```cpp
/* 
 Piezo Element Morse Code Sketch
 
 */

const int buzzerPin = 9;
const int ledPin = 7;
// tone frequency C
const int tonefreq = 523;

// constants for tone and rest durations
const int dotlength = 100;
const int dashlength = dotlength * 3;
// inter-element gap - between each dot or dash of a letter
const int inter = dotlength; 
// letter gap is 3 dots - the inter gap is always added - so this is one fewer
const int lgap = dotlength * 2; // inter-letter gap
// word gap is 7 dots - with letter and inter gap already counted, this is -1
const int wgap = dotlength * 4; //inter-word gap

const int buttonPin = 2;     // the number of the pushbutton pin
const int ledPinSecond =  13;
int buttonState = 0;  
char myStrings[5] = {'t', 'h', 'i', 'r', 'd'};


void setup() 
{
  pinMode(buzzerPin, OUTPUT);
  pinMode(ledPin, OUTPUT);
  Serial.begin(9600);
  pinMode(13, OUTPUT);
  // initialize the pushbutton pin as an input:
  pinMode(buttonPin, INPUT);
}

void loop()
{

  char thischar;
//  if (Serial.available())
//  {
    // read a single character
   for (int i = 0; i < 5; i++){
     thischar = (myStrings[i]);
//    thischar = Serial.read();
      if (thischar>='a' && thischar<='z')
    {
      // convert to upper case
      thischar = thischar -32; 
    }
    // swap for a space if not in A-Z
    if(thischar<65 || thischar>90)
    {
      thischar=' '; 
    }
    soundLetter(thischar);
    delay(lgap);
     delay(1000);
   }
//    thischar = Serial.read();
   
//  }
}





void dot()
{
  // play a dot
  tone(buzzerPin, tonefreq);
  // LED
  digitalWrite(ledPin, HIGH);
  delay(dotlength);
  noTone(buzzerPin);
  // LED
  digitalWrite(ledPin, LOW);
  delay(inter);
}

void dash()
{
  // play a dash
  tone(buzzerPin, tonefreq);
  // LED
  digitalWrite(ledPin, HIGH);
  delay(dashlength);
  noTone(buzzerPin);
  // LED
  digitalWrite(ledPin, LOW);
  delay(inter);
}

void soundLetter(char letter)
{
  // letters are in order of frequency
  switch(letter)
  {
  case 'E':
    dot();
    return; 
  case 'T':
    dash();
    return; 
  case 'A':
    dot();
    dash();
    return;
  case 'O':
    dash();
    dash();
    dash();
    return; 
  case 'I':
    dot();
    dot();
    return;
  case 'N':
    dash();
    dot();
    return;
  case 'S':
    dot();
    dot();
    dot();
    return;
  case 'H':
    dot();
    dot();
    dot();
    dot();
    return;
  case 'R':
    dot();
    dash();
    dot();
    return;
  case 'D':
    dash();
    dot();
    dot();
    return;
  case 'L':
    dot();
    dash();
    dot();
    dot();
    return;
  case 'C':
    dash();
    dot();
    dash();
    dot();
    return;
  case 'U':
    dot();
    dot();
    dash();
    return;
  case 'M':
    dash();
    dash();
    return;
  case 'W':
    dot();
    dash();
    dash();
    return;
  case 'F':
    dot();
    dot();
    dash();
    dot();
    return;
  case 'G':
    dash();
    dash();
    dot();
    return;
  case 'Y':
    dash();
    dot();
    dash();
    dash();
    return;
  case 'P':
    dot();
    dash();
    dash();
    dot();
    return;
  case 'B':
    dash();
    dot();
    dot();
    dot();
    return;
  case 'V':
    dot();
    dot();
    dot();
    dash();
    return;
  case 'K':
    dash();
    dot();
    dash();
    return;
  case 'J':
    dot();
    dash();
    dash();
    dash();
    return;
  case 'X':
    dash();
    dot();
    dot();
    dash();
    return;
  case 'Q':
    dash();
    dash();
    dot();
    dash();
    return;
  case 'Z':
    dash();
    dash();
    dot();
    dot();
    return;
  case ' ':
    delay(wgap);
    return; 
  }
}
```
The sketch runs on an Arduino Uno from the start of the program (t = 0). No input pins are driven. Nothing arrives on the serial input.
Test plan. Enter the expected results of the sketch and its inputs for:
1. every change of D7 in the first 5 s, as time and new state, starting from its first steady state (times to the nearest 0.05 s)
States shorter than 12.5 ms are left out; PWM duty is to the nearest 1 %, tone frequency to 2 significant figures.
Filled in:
0 s high; 0.3 s low; 1.6 s high; 1.7 s low; 1.8 s high; 1.9 s low; 2 s high; 2.1 s low; 2.2 s high; 2.3 s low; 3.6 s high; 3.7 s low; 3.8 s high; 3.9 s low
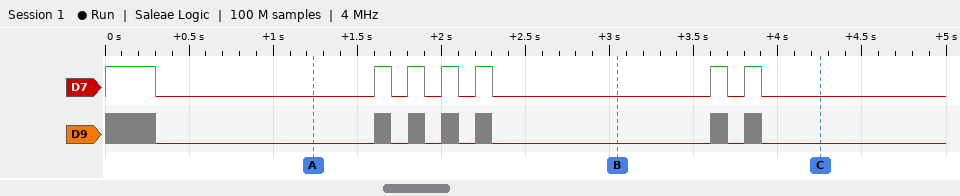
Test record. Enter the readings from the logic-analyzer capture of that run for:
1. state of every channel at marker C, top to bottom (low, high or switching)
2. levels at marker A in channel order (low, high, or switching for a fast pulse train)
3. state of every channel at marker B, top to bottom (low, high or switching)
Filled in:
D7 low, D9 low
D7 low, D9 low
D7 low, D9 low
